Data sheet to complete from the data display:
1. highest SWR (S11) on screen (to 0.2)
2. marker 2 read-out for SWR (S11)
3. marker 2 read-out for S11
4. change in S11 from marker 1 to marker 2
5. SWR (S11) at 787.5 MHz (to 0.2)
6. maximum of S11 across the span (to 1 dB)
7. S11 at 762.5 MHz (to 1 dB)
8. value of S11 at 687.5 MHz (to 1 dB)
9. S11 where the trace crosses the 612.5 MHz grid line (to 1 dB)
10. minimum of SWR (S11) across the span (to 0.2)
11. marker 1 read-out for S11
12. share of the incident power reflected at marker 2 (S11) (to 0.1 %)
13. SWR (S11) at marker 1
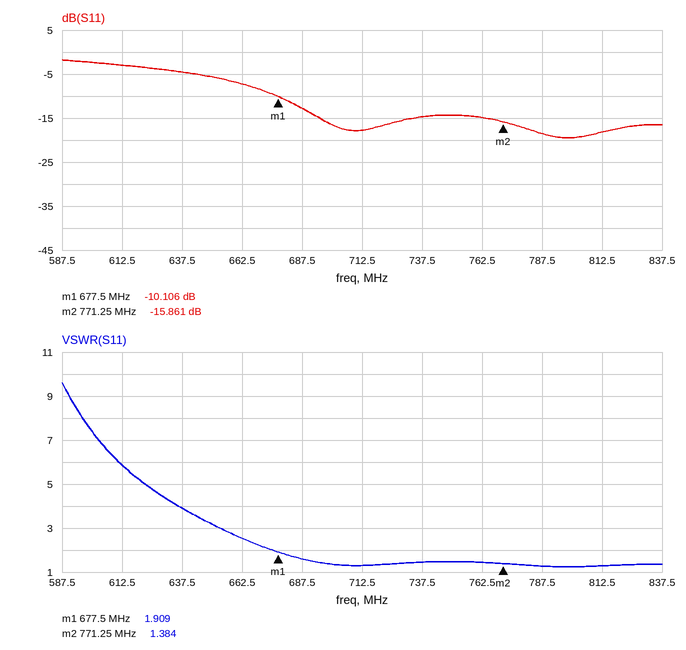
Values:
9.6
1.384
-15.861 dB
-5.755 dB
1.2
-2 dB
-15 dB
-13 dB
-3 dB
1.2
-10.106 dB
2.6 %
1.909
